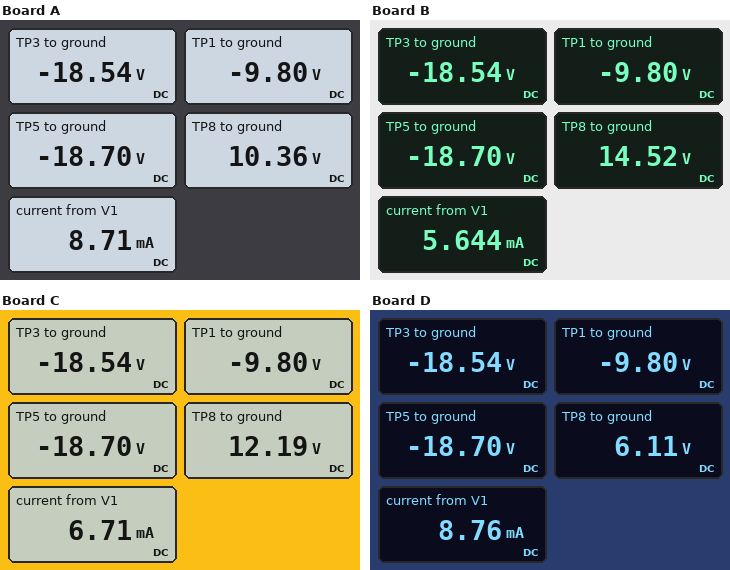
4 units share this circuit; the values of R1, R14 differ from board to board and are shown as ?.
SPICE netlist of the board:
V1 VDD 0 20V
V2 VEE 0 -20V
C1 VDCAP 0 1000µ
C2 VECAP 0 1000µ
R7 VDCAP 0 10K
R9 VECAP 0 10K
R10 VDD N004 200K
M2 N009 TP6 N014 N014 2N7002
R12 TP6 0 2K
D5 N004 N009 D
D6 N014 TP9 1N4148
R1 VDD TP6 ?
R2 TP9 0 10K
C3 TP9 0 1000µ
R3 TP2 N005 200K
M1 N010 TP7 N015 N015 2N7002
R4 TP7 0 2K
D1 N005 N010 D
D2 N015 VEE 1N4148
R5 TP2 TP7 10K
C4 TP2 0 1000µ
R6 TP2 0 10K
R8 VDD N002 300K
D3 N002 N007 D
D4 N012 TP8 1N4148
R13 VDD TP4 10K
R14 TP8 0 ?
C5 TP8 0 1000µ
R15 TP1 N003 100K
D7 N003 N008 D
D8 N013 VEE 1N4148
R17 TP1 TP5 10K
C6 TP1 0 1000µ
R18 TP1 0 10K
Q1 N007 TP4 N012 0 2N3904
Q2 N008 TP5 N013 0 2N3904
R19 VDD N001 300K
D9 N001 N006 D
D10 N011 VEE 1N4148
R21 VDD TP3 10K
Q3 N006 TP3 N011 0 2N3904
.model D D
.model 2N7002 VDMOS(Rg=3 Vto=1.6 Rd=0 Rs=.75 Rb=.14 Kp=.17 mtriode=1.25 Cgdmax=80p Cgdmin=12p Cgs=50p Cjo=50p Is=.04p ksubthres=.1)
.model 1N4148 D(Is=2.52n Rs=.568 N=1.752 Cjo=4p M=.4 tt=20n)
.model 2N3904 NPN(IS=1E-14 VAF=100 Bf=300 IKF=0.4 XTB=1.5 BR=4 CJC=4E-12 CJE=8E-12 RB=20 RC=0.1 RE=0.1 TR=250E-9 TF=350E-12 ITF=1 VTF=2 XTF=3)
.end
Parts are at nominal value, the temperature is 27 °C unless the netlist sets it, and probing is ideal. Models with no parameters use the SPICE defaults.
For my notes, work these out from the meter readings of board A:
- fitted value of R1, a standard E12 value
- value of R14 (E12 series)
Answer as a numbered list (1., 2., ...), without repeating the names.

1. 3.3 kΩ
2. 12 kΩ
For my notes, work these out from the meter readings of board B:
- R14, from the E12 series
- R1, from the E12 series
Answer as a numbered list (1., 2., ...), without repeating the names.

1. 33 kΩ
2. 15 kΩ
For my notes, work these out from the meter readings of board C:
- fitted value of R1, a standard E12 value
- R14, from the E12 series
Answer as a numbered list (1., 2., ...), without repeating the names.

1. 8.2 kΩ
2. 18 kΩ
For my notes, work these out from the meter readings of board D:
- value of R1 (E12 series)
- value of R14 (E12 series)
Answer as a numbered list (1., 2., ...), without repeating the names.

1. 3.9 kΩ
2. 4.7 kΩ
